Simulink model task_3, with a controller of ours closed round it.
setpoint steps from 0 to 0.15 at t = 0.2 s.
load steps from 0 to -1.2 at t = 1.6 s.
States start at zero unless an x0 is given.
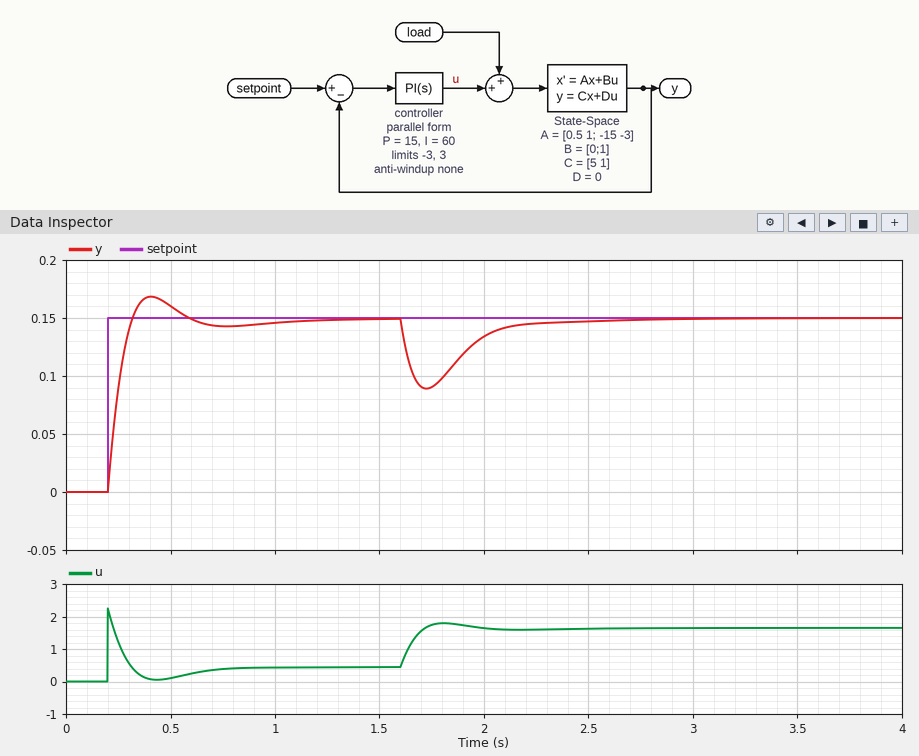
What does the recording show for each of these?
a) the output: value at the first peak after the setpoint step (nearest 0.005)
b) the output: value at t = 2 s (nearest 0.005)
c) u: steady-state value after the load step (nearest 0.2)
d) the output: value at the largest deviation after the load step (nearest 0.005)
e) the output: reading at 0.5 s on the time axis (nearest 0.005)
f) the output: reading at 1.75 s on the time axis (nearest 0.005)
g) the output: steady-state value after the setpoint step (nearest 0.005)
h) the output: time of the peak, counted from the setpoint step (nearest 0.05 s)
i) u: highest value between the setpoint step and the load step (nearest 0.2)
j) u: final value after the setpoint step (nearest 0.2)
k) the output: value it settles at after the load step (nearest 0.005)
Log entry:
0.170
0.135
1.6
0.090
0.160
0.090
0.150
0.20 s
2.2
0.4
0.150
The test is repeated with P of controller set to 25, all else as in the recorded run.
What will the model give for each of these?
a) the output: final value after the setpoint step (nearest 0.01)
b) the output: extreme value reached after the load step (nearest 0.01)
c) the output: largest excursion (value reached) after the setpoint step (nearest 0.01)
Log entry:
0.15
0.11
0.16
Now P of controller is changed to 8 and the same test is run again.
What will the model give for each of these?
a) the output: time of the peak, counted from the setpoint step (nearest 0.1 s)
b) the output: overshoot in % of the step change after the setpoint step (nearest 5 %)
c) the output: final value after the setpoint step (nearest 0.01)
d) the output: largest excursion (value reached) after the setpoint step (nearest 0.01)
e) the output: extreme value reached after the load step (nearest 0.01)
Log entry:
0.3 s
25 %
0.15
0.19
0.06
